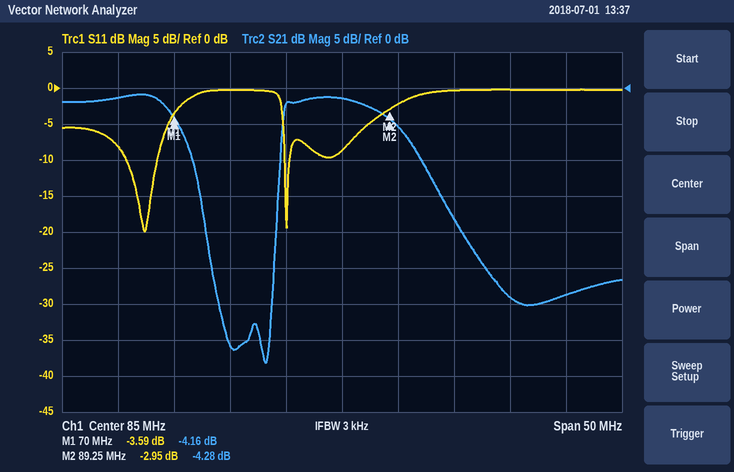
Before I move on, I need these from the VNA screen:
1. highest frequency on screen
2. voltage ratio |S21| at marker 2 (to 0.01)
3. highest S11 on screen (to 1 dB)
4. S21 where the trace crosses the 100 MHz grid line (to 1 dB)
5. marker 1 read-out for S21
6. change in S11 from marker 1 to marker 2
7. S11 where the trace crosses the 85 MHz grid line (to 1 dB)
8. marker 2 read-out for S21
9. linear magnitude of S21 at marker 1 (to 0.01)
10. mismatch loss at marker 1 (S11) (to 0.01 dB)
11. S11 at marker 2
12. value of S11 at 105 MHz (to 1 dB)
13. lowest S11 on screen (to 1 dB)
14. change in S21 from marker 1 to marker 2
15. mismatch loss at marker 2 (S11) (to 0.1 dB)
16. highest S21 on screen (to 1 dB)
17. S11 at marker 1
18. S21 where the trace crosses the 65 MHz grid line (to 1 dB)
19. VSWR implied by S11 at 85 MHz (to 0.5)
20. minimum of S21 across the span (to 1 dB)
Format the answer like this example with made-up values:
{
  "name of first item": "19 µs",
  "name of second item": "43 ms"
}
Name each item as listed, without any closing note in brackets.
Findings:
{
  "highest frequency on screen": "110 MHz",
  "voltage ratio |S21| at marker 2": "0.61",
  "highest S11 on screen": "0 dB",
  "S21 where the trace crosses the 100 MHz grid line": "-29 dB",
  "marker 1 read-out for S21": "-4.16 dB",
  "change in S11 from marker 1 to marker 2": "0.64 dB",
  "S11 where the trace crosses the 85 MHz grid line": "-9 dB",
  "marker 2 read-out for S21": "-4.28 dB",
  "linear magnitude of S21 at marker 1": "0.62",
  "mismatch loss at marker 1 (S11)": "2.50 dB",
  "S11 at marker 2": "-2.95 dB",
  "value of S11 at 105 MHz": "0 dB",
  "lowest S11 on screen": "-20 dB",
  "change in S21 from marker 1 to marker 2": "-0.12 dB",
  "mismatch loss at marker 2 (S11)": "3.1 dB",
  "highest S21 on screen": "-1 dB",
  "S11 at marker 1": "-3.59 dB",
  "S21 where the trace crosses the 65 MHz grid line": "-1 dB",
  "VSWR implied by S11 at 85 MHz": "2.0",
  "minimum of S21 across the span": "-38 dB"
}
